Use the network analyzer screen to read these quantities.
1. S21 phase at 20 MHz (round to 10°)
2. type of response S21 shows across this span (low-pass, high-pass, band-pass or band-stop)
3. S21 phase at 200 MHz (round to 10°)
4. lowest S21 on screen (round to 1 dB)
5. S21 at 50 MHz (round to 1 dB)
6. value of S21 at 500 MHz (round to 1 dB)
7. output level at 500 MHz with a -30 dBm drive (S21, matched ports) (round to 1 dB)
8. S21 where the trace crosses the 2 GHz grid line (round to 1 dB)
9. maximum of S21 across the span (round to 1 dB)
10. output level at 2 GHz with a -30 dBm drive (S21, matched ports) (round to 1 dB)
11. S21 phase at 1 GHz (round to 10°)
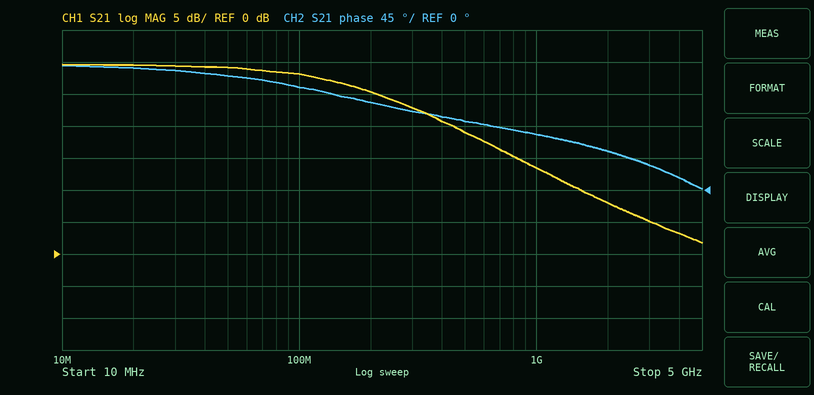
170°
low-pass
120°
2 dB
29 dB
19 dB
-11 dBm
8 dB
30 dB
-22 dBm
80°
